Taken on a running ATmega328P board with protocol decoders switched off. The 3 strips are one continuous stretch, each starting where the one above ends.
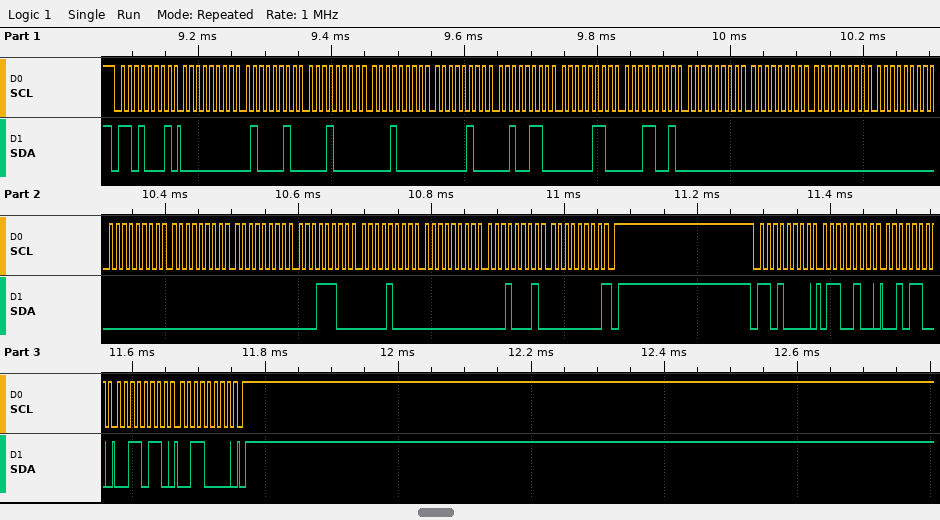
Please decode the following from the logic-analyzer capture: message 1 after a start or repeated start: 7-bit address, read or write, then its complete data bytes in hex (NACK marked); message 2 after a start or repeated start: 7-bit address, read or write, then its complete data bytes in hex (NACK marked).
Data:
0x68 read: 00 42 10 10 04 26 06 19 00 00 00 00 00 00 00 1C 08 00 11 00 NACK
0x68 write: 64 2C 36 30
